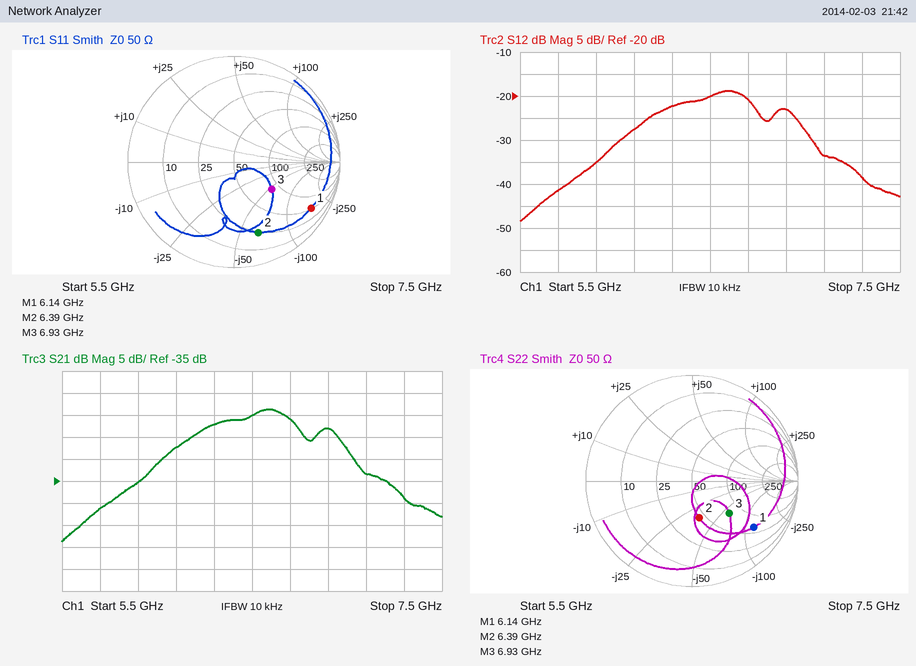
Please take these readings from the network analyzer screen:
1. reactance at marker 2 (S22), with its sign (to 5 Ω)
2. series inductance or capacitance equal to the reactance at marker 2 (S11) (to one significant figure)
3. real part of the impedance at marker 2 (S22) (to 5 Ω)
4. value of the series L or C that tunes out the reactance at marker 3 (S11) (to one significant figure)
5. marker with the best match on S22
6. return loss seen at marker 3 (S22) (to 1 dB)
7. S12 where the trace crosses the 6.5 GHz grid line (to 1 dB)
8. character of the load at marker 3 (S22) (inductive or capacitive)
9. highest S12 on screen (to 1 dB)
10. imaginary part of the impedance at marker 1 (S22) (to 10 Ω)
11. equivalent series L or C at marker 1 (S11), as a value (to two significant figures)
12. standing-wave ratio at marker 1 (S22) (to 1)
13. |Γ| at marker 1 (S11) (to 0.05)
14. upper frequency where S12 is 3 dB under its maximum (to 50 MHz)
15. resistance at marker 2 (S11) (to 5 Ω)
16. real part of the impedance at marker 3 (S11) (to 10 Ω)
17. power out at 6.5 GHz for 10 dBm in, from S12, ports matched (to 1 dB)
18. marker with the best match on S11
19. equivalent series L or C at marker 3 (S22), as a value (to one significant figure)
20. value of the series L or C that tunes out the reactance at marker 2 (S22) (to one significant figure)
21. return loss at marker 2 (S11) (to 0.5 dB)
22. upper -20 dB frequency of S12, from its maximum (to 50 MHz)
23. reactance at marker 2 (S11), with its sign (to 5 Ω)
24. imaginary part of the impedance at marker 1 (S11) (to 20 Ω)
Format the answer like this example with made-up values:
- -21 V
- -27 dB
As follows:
- -35 Ω
- 400 fF
- 45 Ω
- 1 nH
- marker 2
- 7 dB
- -20 dB
- capacitive
- -19 dB
- -120 Ω
- 160 fF
- 6
- 0.85
- 6.70 GHz
- 25 Ω
- 80 Ω
- -10 dBm
- marker 3
- 400 fF
- 900 pH
- 3.0 dB
- 7.30 GHz
- -65 Ω
- -160 Ω
